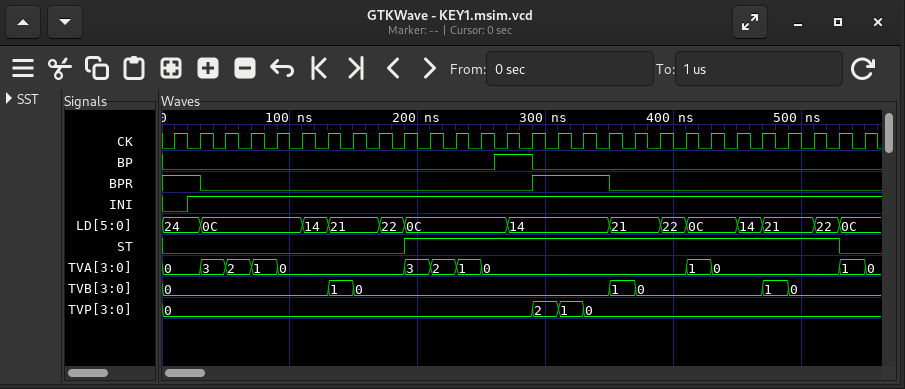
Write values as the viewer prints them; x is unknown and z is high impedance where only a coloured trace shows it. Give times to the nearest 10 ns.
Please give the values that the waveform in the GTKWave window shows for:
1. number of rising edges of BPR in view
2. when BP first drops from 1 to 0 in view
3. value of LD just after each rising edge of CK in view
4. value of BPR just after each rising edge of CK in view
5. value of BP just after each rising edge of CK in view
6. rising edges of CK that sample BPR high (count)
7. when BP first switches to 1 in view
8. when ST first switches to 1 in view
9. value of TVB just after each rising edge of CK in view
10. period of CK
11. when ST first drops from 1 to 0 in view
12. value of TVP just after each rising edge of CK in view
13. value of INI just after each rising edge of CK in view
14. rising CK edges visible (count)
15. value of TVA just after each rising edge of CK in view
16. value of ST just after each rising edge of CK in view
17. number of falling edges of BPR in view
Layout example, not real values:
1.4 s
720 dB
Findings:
1
290 ns
24, 0C, 0C, 0C, 0C, 14, 21, 21, 22, 0C, 0C, 0C, 0C, 14, 14, 14, 14, 21, 21, 22, 0C, 0C, 14, 21, 21, 22, 0C, 0C
1 0 0 0 0 0 0 0 0 0 0 0 0 0 1 1 1 0 0 0 0 0 0 0 0 0 0 0
0 0 0 0 0 0 0 0 0 0 0 0 0 1 0 0 0 0 0 0 0 0 0 0 0 0 0 0
5
260 ns
190 ns
0, 0, 0, 0, 0, 0, 1, 0, 0, 0, 0, 0, 0, 0, 0, 0, 0, 1, 0, 0, 0, 0, 0, 1, 0, 0, 0, 0
20 ns
530 ns
0, 0, 0, 0, 0, 0, 0, 0, 0, 0, 0, 0, 0, 0, 2, 1, 0, 0, 0, 0, 0, 0, 0, 0, 0, 0, 0, 0
0 1 1 1 1 1 1 1 1 1 1 1 1 1 1 1 1 1 1 1 1 1 1 1 1 1 1 1
28
0, 3, 2, 1, 0, 0, 0, 0, 0, 3, 2, 1, 0, 0, 0, 0, 0, 0, 0, 0, 1, 0, 0, 0, 0, 0, 1, 0
0 0 0 0 0 0 0 0 0 1 1 1 1 1 1 1 1 1 1 1 1 1 1 1 1 1 0 0
2
